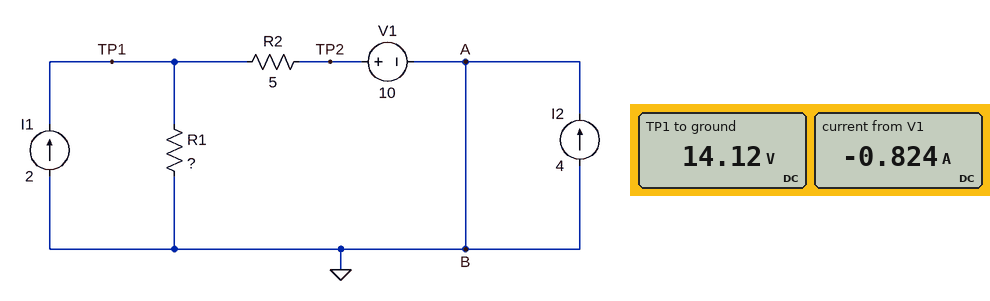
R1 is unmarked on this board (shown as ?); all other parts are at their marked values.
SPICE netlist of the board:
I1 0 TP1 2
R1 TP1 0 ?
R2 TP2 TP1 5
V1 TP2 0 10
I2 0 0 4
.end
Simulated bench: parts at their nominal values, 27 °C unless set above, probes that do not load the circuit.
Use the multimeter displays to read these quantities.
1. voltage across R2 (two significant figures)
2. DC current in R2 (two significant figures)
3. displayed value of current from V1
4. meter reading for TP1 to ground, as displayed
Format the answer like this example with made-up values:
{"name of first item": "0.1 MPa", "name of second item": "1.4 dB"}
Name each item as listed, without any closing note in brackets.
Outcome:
{"voltage across R2": "4.1 V", "DC current in R2": "820 mA", "displayed value of current from V1": "-0.824 A", "meter reading for TP1 to ground, as displayed": "14.12 V"}
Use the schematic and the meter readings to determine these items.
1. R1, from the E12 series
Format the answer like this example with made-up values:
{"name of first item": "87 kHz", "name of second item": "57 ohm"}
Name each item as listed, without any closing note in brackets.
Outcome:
{"R1, from the E12 series": "12 Ω"}
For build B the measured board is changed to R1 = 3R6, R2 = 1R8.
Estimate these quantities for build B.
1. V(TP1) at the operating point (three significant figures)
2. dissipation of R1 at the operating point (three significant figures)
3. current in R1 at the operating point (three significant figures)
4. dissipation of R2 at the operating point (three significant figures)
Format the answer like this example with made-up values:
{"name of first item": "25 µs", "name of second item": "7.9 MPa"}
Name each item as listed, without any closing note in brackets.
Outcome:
{"V(TP1) at the operating point": "9.07 V", "dissipation of R1 at the operating point": "22.8 W", "current in R1 at the operating point": "2.52 A", "dissipation of R2 at the operating point": "484 mW"}
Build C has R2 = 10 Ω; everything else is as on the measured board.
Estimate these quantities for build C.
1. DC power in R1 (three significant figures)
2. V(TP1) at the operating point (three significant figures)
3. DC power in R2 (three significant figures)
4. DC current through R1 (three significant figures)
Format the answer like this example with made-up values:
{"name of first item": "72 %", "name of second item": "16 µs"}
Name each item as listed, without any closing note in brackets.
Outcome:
{"DC power in R1": "22.3 W", "V(TP1) at the operating point": "16.4 V", "DC power in R2": "4.05 W", "DC current through R1": "1.36 A"}
